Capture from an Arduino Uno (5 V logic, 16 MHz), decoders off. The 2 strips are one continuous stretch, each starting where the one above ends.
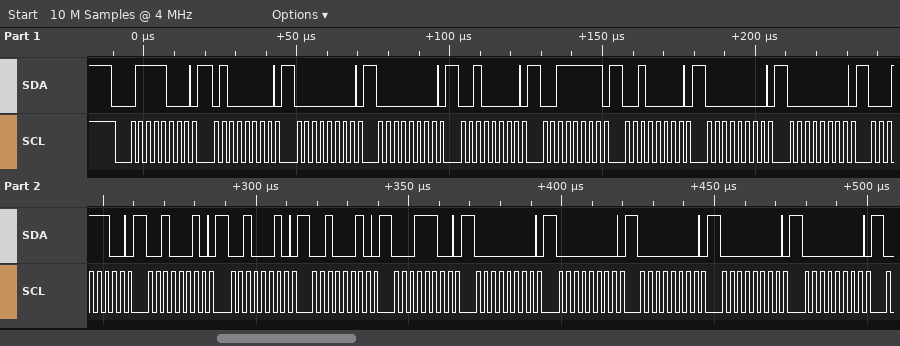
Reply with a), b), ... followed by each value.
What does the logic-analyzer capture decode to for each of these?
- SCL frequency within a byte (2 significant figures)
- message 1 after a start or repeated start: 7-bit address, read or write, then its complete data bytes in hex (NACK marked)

a) 400 kHz
b) 0x3C write: 40 00 00 20 3F 20 00 00 1C 22 22 22 1C 00 00 00 00 00
